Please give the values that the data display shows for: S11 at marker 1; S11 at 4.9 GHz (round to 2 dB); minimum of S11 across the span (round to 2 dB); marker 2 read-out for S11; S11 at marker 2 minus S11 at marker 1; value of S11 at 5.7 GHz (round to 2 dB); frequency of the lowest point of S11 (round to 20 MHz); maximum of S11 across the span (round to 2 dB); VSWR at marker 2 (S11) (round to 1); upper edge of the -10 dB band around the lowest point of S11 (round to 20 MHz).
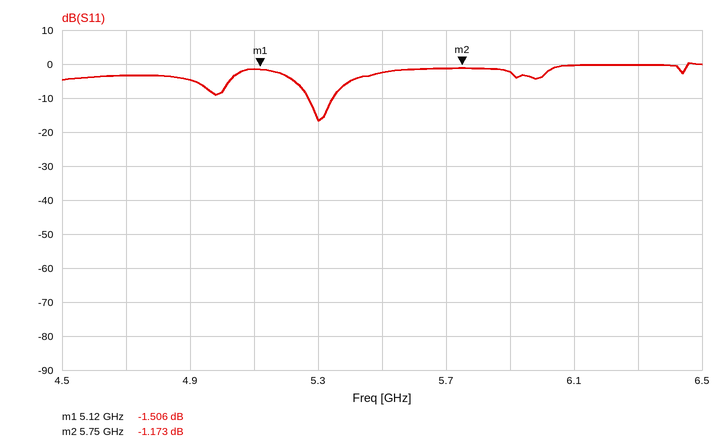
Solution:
-1.506 dB
-4 dB
-16 dB
-1.173 dB
0.333 dB
-2 dB
5.30 GHz
0 dB
15
5.34 GHz
